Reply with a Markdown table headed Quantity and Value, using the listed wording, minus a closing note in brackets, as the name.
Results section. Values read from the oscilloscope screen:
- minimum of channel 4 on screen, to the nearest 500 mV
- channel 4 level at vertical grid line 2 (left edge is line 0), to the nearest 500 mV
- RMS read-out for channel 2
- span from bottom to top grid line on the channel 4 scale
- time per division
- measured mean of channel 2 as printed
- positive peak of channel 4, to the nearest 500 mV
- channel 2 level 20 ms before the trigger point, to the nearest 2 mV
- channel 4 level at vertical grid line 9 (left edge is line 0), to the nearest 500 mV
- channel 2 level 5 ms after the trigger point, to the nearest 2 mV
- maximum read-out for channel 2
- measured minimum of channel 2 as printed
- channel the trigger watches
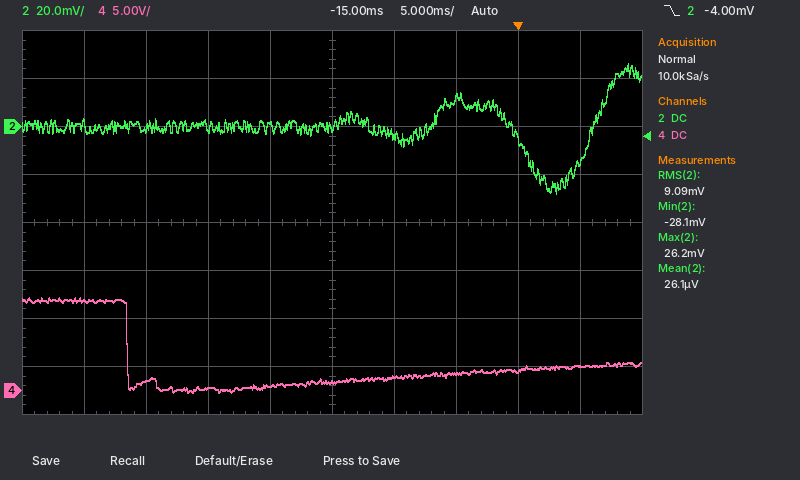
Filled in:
| Quantity | Value |
|---|---|
| minimum of channel 4 on screen, to the nearest 500 mV | 0.0 V |
| channel 4 level at vertical grid line 2 (left edge is line 0), to the nearest 500 mV | 1.0 V |
| RMS read-out for channel 2 | 9.09 mV |
| span from bottom to top grid line on the channel 4 scale | 40 V |
| time per division | 5 ms |
| measured mean of channel 2 as printed | 26.1 µV |
| positive peak of channel 4, to the nearest 500 mV | 9.5 V |
| channel 2 level 20 ms before the trigger point, to the nearest 2 mV | 0 mV |
| channel 4 level at vertical grid line 9 (left edge is line 0), to the nearest 500 mV | 2.5 V |
| channel 2 level 5 ms after the trigger point, to the nearest 2 mV | -14 mV |
| maximum read-out for channel 2 | 26.2 mV |
| measured minimum of channel 2 as printed | -28.1 mV |
| channel the trigger watches | channel 2 |
